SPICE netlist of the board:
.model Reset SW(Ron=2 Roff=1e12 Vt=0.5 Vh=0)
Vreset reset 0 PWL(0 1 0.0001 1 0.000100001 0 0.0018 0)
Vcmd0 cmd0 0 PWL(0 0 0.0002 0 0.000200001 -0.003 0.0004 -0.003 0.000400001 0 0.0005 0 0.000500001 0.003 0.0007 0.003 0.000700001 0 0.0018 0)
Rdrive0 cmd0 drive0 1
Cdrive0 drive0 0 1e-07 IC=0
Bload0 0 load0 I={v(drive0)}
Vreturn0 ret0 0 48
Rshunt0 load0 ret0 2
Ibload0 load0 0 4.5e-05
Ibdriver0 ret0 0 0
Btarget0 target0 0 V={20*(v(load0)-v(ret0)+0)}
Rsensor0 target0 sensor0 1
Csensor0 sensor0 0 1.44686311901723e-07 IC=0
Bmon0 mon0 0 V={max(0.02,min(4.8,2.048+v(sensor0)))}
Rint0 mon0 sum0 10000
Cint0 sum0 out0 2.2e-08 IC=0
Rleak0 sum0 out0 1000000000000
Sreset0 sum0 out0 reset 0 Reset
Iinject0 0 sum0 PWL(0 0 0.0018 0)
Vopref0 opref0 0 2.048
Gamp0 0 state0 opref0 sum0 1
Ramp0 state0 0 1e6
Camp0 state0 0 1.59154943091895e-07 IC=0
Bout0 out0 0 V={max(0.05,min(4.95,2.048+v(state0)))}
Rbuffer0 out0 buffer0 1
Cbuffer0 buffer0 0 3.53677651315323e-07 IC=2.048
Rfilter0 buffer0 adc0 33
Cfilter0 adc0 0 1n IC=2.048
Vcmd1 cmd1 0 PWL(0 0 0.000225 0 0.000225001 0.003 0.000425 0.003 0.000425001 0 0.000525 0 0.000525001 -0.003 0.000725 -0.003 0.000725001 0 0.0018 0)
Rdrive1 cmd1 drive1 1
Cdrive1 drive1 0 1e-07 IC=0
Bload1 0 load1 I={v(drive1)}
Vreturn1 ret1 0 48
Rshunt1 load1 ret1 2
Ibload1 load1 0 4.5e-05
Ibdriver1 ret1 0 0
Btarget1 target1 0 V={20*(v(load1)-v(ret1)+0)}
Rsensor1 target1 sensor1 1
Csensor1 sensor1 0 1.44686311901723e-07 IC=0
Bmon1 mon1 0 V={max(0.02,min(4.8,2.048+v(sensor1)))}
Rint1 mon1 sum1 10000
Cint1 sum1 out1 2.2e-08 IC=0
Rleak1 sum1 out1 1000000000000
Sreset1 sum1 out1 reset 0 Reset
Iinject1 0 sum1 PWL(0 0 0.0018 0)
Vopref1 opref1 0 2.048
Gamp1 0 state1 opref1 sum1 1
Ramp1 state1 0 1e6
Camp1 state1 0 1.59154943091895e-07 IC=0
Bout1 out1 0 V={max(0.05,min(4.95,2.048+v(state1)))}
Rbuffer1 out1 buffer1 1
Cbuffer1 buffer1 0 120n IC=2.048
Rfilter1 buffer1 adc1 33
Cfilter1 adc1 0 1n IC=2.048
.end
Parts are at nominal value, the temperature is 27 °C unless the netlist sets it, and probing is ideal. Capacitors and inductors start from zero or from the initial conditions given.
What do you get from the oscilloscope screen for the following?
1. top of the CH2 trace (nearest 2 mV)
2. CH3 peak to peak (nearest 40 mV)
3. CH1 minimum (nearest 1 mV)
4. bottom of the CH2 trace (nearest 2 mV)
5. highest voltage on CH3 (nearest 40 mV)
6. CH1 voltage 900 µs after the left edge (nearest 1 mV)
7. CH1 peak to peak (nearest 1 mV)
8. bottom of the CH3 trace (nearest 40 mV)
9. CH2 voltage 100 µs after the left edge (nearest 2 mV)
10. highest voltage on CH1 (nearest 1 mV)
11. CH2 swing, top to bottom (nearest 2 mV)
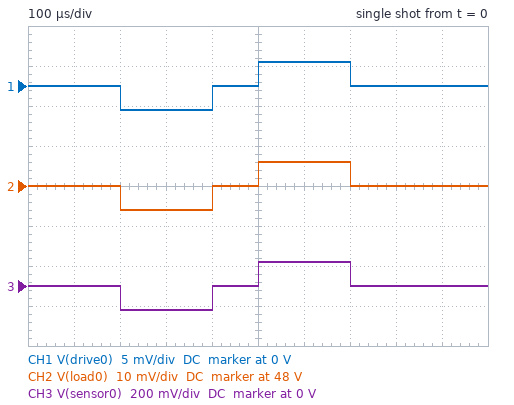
48.006 V
240 mV
-3 mV
47.994 V
120 mV
0 V
6 mV
-120 mV
48.000 V
3 mV
12 mV
